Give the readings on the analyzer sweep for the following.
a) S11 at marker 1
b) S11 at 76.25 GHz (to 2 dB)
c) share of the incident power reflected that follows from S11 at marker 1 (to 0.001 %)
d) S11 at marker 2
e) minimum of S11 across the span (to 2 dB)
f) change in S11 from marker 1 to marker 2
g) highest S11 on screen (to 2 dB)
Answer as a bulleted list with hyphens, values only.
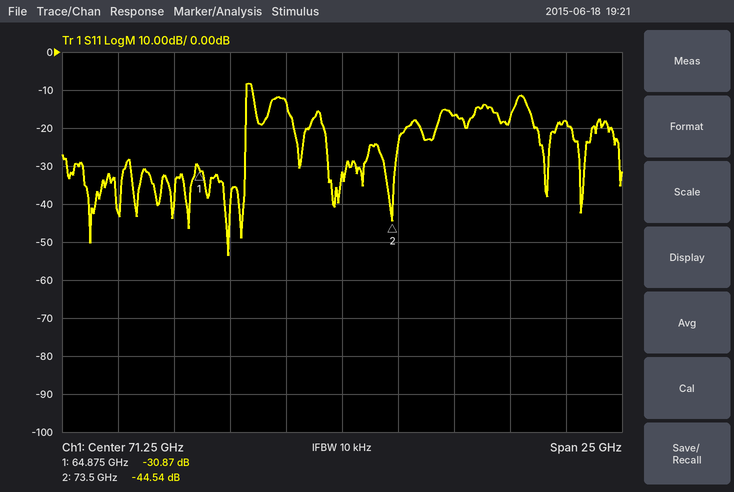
- -30.87 dB
- -16 dB
- 0.082 %
- -44.54 dB
- -54 dB
- -13.67 dB
- -8 dB
